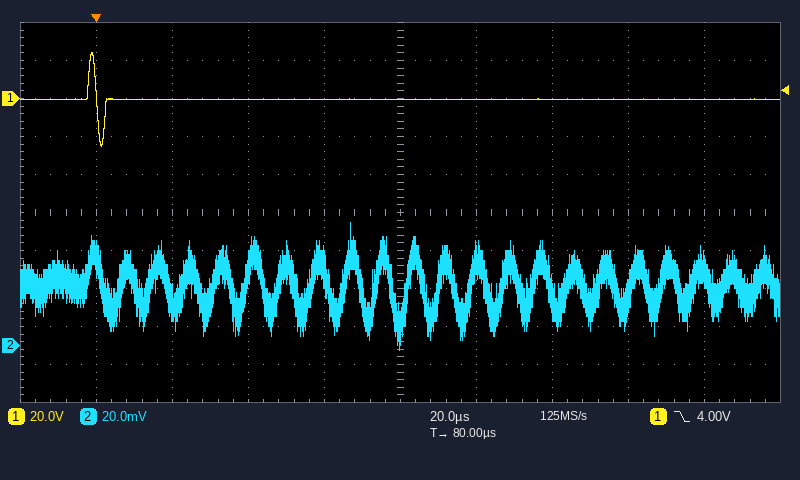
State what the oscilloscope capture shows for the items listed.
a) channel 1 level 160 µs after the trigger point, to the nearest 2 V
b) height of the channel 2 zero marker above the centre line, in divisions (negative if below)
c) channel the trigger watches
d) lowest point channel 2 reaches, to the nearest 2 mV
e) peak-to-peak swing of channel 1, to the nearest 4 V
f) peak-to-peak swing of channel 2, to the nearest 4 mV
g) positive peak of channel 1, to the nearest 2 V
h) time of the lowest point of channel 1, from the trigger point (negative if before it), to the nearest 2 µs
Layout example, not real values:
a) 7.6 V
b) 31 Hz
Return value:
a) 0 V
b) -3.5 div
c) channel 1
d) -2 mV
e) 48 V
f) 68 mV
g) 24 V
h) +2 µs
